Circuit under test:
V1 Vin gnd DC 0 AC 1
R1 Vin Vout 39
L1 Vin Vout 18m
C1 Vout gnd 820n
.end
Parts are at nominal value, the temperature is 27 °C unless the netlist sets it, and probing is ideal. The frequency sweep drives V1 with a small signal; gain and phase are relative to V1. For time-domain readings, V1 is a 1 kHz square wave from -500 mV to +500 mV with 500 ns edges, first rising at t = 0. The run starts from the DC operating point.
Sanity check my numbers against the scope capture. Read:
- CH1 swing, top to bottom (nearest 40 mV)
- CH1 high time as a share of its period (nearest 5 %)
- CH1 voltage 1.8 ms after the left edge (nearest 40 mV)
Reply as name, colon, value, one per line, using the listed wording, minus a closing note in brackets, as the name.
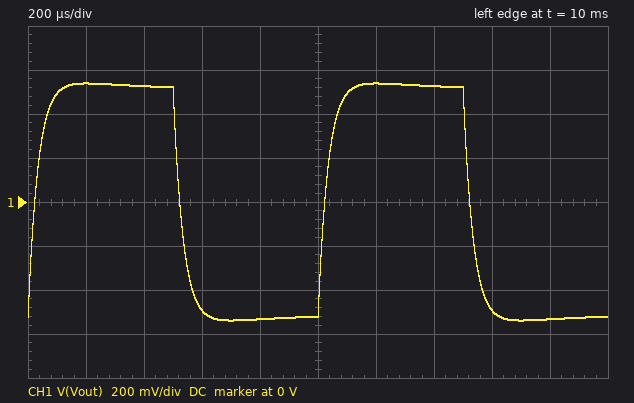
CH1 swing, top to bottom: 1.08 V
CH1 high time as a share of its period: 50 %
CH1 voltage 1.8 ms after the left edge: -520 mV
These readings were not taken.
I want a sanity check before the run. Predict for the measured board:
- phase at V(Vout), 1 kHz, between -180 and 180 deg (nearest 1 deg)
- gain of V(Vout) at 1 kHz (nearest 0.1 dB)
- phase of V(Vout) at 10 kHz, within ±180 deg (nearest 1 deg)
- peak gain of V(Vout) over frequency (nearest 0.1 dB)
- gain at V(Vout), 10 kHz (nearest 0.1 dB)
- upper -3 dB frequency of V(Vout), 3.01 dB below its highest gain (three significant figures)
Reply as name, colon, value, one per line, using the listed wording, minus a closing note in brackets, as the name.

phase at V(Vout), 1 kHz, between -180 and 180 deg: -11 deg
gain of V(Vout) at 1 kHz: 0.4 dB
phase of V(Vout) at 10 kHz, within ±180 deg: -65 deg
peak gain of V(Vout) over frequency: 0.4 dB
gain at V(Vout), 10 kHz: -6.9 dB
upper -3 dB frequency of V(Vout), 3.01 dB below its highest gain: 4.85 kHz
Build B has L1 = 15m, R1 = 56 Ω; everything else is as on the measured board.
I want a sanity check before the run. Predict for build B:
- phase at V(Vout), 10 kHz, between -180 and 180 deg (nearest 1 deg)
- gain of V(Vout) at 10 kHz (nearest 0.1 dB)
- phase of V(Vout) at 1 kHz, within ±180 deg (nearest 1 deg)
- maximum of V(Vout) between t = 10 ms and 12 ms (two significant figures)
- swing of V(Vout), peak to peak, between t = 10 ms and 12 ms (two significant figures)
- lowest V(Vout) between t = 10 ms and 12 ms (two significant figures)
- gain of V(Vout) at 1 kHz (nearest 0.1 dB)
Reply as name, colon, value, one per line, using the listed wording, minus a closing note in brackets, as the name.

phase at V(Vout), 10 kHz, between -180 and 180 deg: -74 deg
gain of V(Vout) at 10 kHz: -9.5 dB
phase of V(Vout) at 1 kHz, within ±180 deg: -14 deg
maximum of V(Vout) between t = 10 ms and 12 ms: 590 mV
swing of V(Vout), peak to peak, between t = 10 ms and 12 ms: 1.2 V
lowest V(Vout) between t = 10 ms and 12 ms: -590 mV
gain of V(Vout) at 1 kHz: 0.9 dB
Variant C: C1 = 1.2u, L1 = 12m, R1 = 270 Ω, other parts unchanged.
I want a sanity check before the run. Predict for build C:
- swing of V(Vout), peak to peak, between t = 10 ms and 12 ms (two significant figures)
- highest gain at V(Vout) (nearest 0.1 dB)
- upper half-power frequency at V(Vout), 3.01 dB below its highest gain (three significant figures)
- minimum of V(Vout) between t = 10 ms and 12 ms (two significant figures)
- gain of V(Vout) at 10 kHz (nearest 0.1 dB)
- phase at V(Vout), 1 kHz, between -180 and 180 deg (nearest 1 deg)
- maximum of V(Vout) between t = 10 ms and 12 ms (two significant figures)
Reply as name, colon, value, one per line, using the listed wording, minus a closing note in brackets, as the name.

swing of V(Vout), peak to peak, between t = 10 ms and 12 ms: 2.6 V
highest gain at V(Vout): 9.3 dB
upper half-power frequency at V(Vout), 3.01 dB below its highest gain: 1.52 kHz
minimum of V(Vout) between t = 10 ms and 12 ms: -1.3 V
gain of V(Vout) at 10 kHz: -25.5 dB
phase at V(Vout), 1 kHz, between -180 and 180 deg: -17 deg
maximum of V(Vout) between t = 10 ms and 12 ms: 1.3 V
